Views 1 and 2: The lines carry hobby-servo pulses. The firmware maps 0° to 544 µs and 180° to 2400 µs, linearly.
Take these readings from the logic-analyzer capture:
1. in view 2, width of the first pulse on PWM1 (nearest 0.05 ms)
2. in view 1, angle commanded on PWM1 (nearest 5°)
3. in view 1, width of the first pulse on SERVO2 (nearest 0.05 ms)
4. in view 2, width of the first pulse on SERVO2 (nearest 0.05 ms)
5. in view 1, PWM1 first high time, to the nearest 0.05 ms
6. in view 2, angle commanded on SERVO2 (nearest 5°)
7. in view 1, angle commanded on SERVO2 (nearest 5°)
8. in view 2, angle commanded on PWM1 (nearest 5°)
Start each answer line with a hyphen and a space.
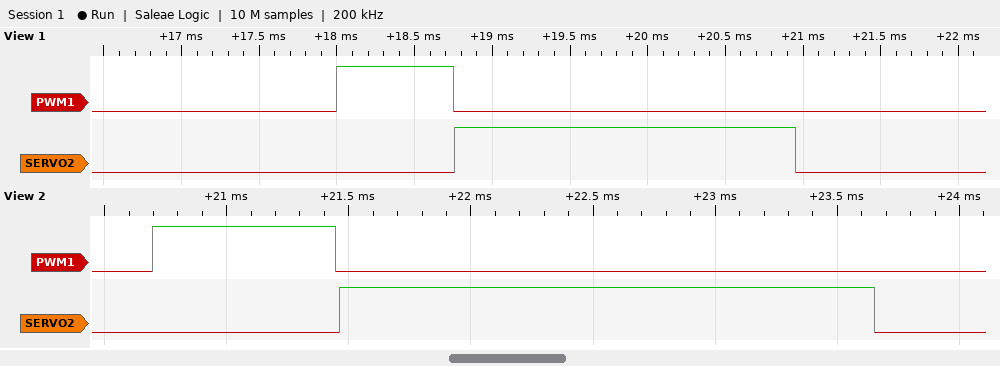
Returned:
- 0.75 ms
- 20°
- 2.20 ms
- 2.20 ms
- 0.75 ms
- 160°
- 160°
- 20°
